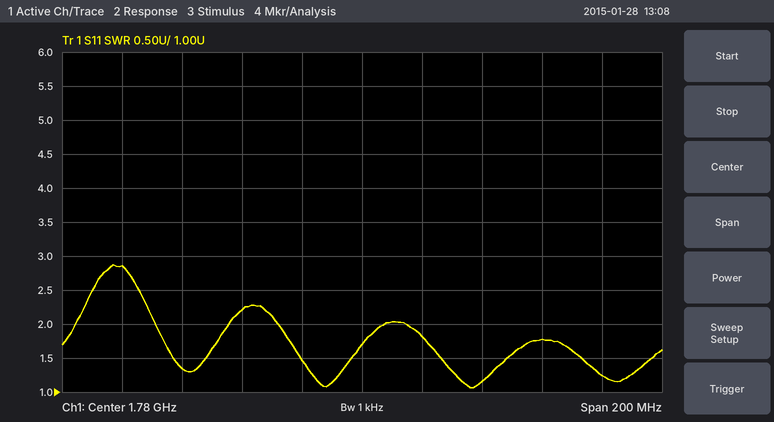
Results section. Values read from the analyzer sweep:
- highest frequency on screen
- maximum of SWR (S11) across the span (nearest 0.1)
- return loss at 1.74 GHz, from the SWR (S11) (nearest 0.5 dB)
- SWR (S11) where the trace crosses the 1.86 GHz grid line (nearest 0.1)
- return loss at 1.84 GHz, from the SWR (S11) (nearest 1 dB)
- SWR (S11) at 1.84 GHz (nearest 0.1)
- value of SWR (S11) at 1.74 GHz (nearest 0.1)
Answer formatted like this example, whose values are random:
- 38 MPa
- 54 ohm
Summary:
- 1.88 GHz
- 2.9
- 8.5 dB
- 1.2
- 11 dB
- 1.8
- 2.2
